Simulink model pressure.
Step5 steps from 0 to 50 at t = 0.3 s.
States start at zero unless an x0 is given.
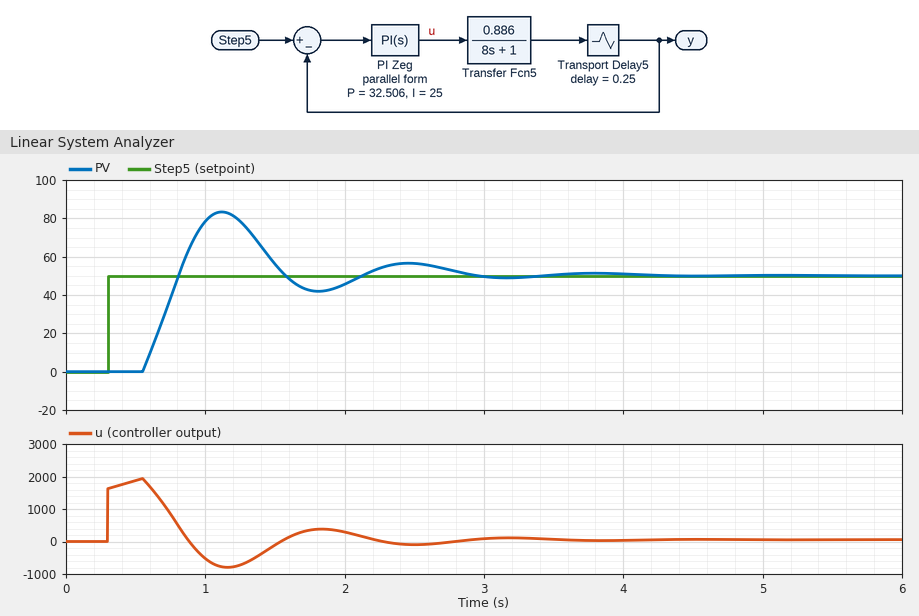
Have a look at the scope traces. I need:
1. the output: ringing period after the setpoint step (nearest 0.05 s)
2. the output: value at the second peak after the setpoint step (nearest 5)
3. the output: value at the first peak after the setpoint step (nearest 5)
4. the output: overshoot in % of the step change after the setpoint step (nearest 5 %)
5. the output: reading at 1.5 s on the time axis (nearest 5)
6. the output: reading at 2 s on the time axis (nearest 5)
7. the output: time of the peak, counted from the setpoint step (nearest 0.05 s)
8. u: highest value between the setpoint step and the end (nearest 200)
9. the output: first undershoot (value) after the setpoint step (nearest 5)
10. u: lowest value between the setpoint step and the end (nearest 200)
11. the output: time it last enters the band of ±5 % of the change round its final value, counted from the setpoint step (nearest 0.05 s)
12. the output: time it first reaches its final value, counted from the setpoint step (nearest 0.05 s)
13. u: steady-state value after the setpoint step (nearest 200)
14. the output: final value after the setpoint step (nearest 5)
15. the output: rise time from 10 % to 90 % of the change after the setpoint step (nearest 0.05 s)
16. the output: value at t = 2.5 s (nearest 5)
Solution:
1.35 s
55
85
65 %
55
45
0.80 s
2000
40
-800
2.50 s
0.50 s
0
50
0.20 s
55
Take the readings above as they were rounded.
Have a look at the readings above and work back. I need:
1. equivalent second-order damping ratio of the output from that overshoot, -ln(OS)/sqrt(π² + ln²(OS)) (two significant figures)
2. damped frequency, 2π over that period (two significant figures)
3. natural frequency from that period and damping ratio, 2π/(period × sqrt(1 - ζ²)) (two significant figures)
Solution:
0.14
4.7 rad/s
4.7 rad/s
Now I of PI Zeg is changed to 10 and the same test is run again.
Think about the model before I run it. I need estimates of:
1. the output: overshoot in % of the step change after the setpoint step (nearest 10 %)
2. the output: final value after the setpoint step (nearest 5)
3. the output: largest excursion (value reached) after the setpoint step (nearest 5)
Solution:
50 %
50
75
